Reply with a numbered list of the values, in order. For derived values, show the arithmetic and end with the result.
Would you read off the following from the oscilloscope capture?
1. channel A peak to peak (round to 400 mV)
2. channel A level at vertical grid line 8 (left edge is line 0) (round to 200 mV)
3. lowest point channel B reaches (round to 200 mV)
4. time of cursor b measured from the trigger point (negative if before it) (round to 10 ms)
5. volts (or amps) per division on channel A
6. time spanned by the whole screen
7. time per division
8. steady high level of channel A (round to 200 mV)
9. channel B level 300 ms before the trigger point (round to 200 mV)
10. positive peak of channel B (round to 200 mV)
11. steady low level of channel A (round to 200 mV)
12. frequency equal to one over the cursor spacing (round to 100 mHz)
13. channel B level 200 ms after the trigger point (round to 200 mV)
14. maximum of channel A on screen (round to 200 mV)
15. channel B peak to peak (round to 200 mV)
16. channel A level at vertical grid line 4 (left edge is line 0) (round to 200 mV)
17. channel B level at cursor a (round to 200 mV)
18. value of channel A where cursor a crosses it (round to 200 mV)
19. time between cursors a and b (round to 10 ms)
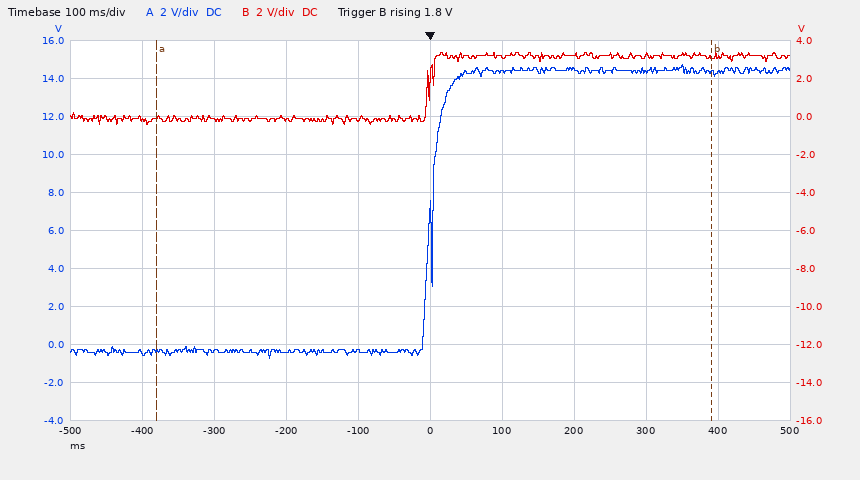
1. 15.6 V
2. 14.4 V
3. -400 mV
4. +390 ms
5. 2 V
6. 1 s
7. 100 ms
8. 14.4 V
9. -200 mV
10. 3.4 V
11. -400 mV
12. 1 / 770 ms ≈ 1.3 Hz
13. 3.2 V
14. 14.8 V
15. 3.4 V − (-400 mV) = 3.8 V
16. -400 mV
17. 0.0 V
18. -400 mV
19. 770 ms
